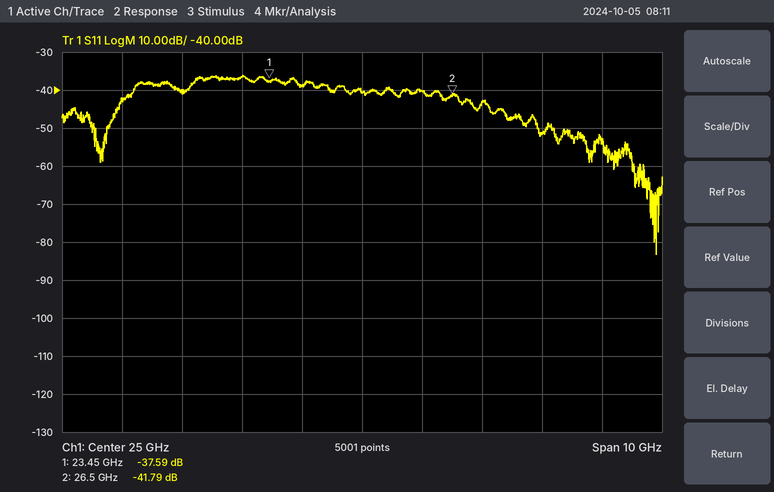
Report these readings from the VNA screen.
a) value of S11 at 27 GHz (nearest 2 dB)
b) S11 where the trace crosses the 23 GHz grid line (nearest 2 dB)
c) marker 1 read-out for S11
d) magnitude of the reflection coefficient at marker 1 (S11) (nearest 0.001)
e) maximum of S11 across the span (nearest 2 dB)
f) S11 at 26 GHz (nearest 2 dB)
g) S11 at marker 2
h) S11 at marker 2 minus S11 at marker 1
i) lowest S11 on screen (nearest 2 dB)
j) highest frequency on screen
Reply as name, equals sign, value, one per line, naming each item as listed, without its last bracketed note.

value of S11 at 27 GHz = -44 dB
S11 where the trace crosses the 23 GHz grid line = -36 dB
marker 1 read-out for S11 = -37.59 dB
magnitude of the reflection coefficient at marker 1 (S11) = 0.013
maximum of S11 across the span = -36 dB
S11 at 26 GHz = -40 dB
S11 at marker 2 = -41.79 dB
S11 at marker 2 minus S11 at marker 1 = -4.20 dB
lowest S11 on screen = -84 dB
highest frequency on screen = 30 GHz
